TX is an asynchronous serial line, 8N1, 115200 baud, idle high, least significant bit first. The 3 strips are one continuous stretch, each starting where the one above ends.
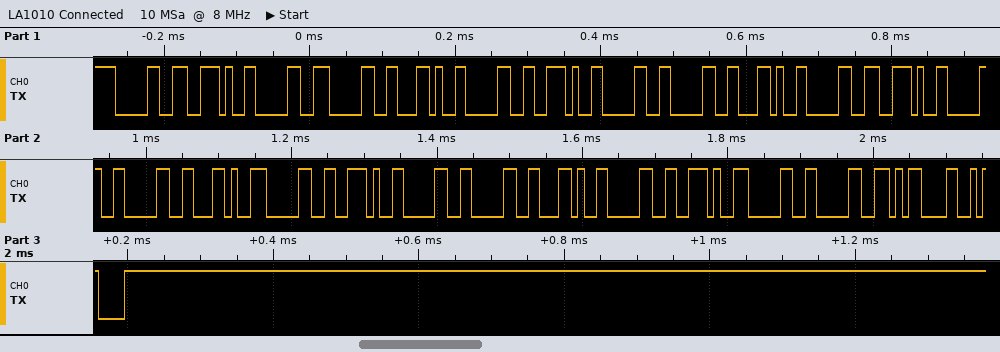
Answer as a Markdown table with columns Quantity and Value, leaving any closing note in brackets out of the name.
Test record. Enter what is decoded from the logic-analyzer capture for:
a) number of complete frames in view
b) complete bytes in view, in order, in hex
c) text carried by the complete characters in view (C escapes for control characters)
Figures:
| Quantity | Value |
|---|---|
| number of complete frames in view | 26 |
| complete bytes in view, in order, in hex | 30 2E 30 30 2C 30 2E 30 30 2C 30 2E 30 30 2C 30 2E 30 30 2C 30 2E 30 30 0D 0A |
| text carried by the complete characters in view | "0.00,0.00,0.00,0.00,0.00\r\n" |
